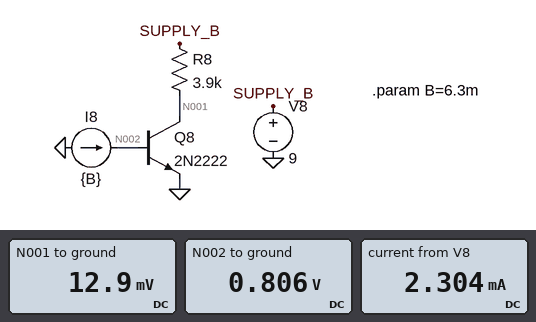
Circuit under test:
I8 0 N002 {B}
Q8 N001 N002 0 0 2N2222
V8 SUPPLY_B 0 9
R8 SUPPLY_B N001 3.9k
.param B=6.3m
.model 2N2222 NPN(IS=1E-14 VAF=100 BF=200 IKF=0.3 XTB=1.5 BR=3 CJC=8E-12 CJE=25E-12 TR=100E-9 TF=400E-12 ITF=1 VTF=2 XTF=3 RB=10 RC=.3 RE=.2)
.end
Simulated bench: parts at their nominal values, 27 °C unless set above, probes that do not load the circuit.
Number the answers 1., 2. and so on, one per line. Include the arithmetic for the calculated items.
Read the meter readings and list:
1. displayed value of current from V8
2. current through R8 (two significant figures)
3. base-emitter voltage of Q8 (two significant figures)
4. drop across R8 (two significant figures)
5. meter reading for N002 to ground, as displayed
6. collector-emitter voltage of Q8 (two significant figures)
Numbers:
1. 2.304 mA
2. (9 V - 12.9 mV) / 3.9 kΩ = 2.3 mA
3. 806 mV = 810 mV
4. 9 V - 12.9 mV = 9.0 V
5. 0.806 V
6. 12.9 mV = 13 mV
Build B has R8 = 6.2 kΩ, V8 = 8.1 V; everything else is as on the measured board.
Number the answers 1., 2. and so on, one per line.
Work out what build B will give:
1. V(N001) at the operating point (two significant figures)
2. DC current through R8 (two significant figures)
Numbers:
1. 11 mV
2. 1.3 mA
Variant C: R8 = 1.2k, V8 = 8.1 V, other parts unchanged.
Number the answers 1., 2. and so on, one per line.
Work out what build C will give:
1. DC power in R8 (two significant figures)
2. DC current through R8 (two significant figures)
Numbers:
1. 54 mW
2. 6.7 mA
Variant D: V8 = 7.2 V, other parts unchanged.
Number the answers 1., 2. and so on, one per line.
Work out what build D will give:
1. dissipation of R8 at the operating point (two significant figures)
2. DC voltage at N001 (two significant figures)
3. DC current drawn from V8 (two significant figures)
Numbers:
1. 13 mW
2. 12 mV
3. 1.8 mA
